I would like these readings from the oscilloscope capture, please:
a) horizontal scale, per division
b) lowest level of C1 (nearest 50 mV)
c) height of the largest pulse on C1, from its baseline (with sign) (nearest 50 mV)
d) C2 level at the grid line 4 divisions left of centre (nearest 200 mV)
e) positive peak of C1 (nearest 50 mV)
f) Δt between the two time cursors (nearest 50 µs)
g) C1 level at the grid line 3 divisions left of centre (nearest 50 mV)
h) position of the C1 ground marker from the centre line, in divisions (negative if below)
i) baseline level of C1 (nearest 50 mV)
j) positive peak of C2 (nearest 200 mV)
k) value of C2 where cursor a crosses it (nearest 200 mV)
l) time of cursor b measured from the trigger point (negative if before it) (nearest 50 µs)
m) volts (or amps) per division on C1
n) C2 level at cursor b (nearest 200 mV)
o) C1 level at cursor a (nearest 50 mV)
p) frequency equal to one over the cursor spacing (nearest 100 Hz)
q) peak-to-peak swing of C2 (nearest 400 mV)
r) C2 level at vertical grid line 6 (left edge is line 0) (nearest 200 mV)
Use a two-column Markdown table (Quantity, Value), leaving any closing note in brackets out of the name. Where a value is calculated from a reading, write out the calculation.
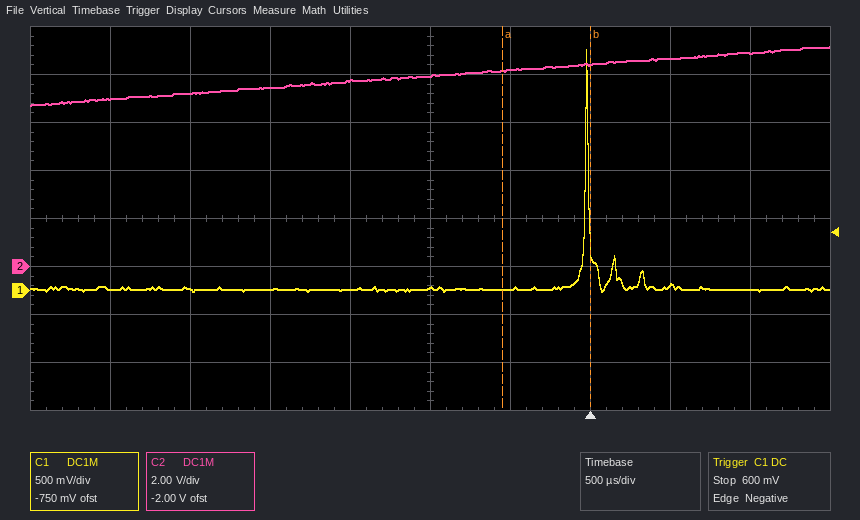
| Quantity | Value |
|---|---|
| horizontal scale, per division | 500 µs |
| lowest level of C1 | 0 mV |
| height of the largest pulse on C1, from its baseline (with sign) | 2.50 V − (0 mV) = +2.50 V |
| C2 level at the grid line 4 divisions left of centre | 7.0 V |
| positive peak of C1 | 2.50 V |
| Δt between the two time cursors | 550 µs |
| C1 level at the grid line 3 divisions left of centre | 0 mV |
| position of the C1 ground marker from the centre line, in divisions | -1.5 div |
| baseline level of C1 | 0 mV |
| positive peak of C2 | 9.2 V |
| value of C2 where cursor a crosses it | 8.2 V |
| time of cursor b measured from the trigger point (negative if before it) | 0 µs |
| volts (or amps) per division on C1 | 500 mV |
| C2 level at cursor b | 8.4 V |
| C1 level at cursor a | 0 mV |
| frequency equal to one over the cursor spacing | 1 / 550 µs ≈ 1.8 kHz |
| peak-to-peak swing of C2 | 2.4 V |
| C2 level at vertical grid line 6 (left edge is line 0) | 8.2 V |
